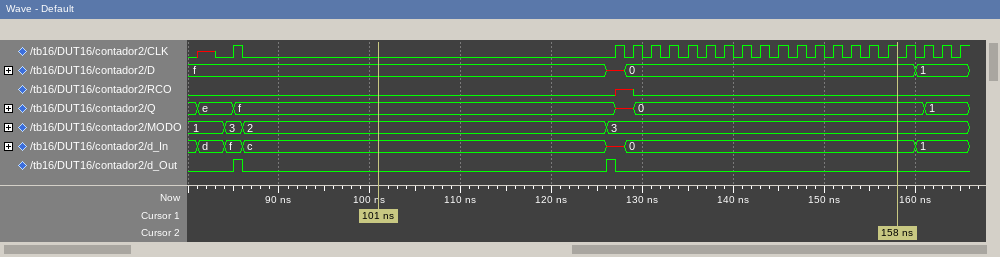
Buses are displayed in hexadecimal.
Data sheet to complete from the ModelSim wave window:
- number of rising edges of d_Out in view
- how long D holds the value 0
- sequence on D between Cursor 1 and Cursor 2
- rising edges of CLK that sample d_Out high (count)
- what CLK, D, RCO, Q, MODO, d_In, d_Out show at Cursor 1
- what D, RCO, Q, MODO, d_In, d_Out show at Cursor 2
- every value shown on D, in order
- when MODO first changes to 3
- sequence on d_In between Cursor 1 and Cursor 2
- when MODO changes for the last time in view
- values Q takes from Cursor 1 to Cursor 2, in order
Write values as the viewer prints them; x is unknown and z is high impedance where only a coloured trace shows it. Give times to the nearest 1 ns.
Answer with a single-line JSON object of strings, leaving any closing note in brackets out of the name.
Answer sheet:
{"number of rising edges of d_Out in view": "2", "how long D holds the value 0": "32 ns", "sequence on D between Cursor 1 and Cursor 2": "f, x, 0", "rising edges of CLK that sample d_Out high": "1", "what CLK, D, RCO, Q, MODO, d_In, d_Out show at Cursor 1": "CLK=0, D=f, RCO=0, Q=f, MODO=2, d_In=c, d_Out=0", "what D, RCO, Q, MODO, d_In, d_Out show at Cursor 2": "D=0, RCO=0, Q=0, MODO=3, d_In=0, d_Out=0", "every value shown on D, in order": "f, x, 0, 1", "when MODO first changes to 3": "84 ns", "sequence on d_In between Cursor 1 and Cursor 2": "c, x, 0", "when MODO changes for the last time in view": "126 ns", "values Q takes from Cursor 1 to Cursor 2, in order": "f, x, 0"}
